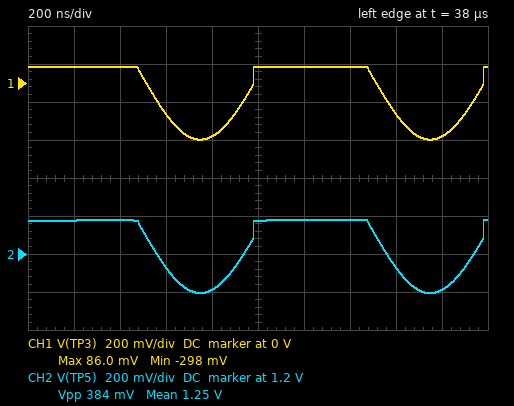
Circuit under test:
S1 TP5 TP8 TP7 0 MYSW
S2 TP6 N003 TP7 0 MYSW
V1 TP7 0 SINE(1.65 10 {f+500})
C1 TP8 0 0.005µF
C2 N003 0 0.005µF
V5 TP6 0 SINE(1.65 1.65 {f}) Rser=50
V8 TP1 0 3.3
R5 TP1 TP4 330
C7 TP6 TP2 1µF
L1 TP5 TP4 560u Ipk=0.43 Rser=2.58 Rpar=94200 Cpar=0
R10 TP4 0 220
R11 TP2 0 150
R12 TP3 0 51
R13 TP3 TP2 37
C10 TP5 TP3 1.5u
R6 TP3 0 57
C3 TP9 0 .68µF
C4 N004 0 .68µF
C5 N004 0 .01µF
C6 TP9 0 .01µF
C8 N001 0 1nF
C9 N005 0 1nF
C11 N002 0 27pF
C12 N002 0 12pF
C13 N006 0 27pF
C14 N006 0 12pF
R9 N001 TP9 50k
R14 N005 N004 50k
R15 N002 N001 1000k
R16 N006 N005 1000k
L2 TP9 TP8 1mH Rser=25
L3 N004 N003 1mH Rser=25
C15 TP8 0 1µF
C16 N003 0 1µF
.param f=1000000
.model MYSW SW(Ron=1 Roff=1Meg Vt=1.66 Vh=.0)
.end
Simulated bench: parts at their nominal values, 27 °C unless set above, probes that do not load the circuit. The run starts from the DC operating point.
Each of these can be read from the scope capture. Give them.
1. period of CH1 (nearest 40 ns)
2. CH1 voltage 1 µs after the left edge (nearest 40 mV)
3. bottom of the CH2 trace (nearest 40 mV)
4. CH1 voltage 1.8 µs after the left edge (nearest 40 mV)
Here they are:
1.00 µs
80 mV
1.00 V
-280 mV
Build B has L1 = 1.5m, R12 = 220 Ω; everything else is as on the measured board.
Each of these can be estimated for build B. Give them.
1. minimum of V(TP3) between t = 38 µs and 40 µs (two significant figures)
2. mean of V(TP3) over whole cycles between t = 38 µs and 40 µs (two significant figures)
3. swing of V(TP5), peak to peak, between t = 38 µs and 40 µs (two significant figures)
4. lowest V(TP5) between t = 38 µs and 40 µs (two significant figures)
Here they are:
-420 mV
-76 mV
520 mV
870 mV
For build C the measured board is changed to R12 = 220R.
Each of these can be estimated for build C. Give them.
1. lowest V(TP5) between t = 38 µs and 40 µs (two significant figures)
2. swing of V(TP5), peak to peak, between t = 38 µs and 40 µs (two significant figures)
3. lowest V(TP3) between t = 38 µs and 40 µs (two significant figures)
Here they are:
870 mV
520 mV
-420 mV
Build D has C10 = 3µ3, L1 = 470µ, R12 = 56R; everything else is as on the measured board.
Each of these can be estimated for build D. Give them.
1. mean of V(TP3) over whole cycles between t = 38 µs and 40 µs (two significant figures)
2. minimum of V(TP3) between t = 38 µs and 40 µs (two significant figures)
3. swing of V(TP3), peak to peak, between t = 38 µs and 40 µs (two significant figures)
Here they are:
-54 mV
-310 mV
390 mV
